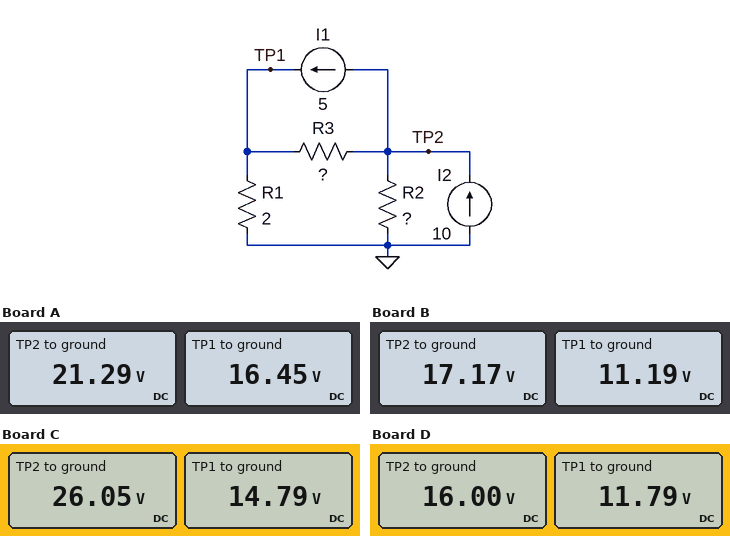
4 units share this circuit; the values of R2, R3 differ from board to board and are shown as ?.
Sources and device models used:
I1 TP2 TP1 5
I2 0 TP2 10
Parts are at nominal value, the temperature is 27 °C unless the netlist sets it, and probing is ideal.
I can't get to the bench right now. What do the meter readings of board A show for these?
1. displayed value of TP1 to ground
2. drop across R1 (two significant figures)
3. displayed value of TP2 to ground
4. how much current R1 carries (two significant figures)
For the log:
16.45 V
16 V
21.29 V
8.2 A
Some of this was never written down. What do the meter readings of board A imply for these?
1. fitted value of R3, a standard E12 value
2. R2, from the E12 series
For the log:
1.5 Ω
12 Ω
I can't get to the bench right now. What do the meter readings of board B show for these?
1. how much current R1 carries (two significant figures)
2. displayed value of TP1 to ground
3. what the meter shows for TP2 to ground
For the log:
5.6 A
11.19 V
17.17 V
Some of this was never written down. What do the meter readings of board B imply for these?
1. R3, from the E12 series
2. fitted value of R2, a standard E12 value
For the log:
10 Ω
3.9 Ω
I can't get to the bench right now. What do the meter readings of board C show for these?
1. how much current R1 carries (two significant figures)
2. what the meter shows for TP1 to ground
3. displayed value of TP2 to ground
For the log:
7.4 A
14.79 V
26.05 V
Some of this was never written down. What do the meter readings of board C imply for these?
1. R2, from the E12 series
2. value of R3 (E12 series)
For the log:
10 Ω
4.7 Ω
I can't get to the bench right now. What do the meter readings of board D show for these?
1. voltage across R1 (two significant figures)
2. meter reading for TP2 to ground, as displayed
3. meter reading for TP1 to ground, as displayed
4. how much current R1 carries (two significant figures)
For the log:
12 V
16.00 V
11.79 V
5.9 A
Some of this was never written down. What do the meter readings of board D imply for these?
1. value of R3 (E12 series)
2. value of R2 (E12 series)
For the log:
4.7 Ω
3.9 Ω
